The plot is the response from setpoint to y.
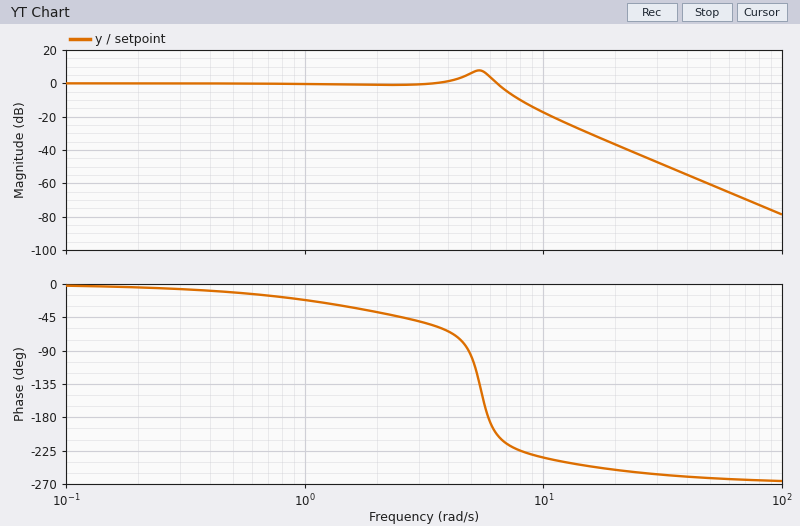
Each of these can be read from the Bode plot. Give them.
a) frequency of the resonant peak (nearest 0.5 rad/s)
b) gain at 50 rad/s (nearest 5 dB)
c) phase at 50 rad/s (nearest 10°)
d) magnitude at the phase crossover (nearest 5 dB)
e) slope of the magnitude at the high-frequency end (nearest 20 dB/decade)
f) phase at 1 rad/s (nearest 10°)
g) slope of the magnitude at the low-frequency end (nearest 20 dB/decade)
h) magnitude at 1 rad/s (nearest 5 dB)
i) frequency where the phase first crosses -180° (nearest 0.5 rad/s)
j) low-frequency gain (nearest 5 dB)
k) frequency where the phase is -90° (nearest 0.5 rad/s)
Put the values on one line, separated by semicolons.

5.5 rad/s; -60 dB; -260°; 5 dB; -60 dB/decade; -20°; 0 dB/decade; 0 dB; 6.0 rad/s; 0 dB; 5.0 rad/s
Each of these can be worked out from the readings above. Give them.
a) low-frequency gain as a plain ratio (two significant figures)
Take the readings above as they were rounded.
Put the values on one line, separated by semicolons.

1.0
